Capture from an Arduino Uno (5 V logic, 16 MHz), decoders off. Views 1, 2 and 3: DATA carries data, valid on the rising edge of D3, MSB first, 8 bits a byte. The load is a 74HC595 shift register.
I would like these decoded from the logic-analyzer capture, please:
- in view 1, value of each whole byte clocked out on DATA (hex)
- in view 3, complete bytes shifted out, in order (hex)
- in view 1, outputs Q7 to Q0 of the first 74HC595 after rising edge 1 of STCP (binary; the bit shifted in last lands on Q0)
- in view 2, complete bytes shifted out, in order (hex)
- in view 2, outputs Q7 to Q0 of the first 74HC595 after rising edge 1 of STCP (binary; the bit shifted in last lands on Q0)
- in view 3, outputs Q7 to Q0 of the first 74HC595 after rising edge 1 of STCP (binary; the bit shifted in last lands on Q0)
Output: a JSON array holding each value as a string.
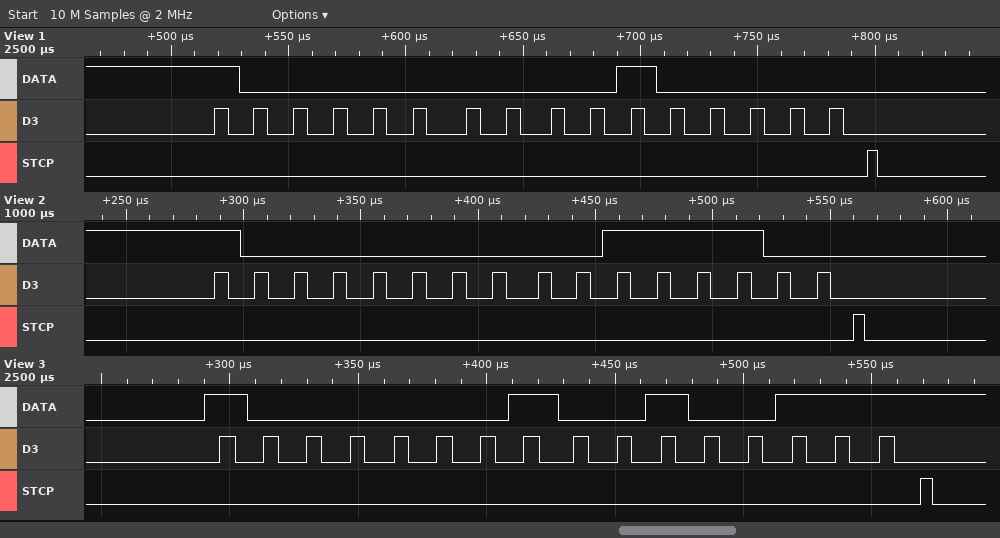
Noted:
["80 20", "0x81 0x27", "00100000", "80 3C", "00111100", "00100111"]
